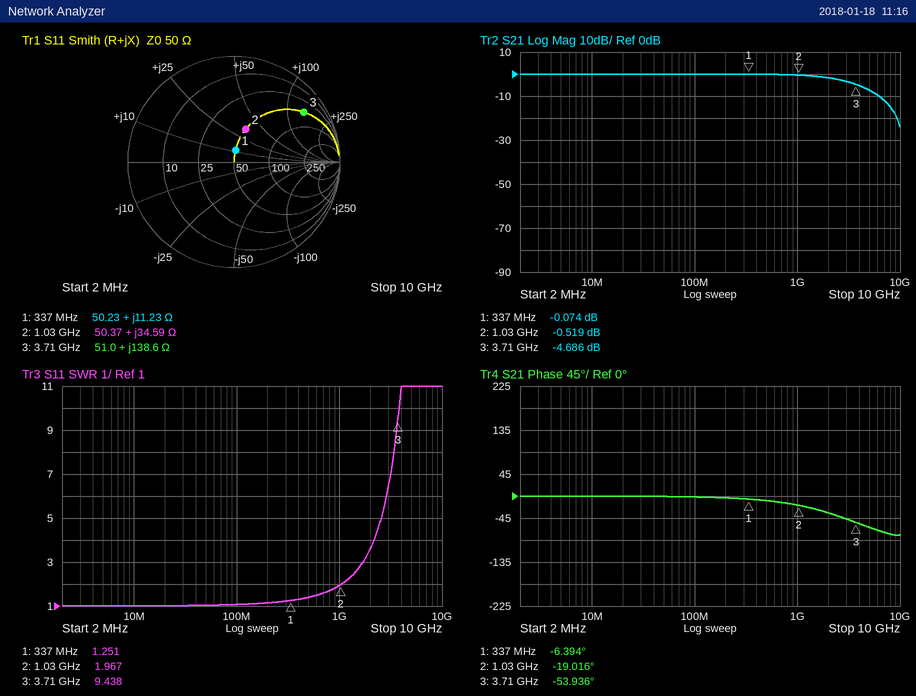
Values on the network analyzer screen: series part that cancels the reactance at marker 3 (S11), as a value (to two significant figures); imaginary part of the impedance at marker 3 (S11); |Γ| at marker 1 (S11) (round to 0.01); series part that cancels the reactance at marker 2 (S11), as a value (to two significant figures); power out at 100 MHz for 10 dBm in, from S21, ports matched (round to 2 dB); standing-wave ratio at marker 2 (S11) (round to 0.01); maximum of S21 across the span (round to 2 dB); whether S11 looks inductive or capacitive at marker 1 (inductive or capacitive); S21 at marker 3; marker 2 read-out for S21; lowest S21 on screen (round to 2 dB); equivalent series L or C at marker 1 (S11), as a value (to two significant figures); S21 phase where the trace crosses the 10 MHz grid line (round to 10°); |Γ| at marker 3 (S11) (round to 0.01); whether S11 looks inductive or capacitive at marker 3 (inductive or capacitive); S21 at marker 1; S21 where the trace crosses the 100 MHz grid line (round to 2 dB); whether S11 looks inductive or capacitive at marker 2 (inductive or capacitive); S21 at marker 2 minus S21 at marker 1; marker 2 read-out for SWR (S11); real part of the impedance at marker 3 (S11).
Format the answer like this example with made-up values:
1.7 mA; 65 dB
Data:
310 fF; +138.6 Ω; 0.11; 4.5 pF; 10 dBm; 1.97; 0 dB; inductive; -4.686 dB; -0.519 dB; -24 dB; 5.3 nH; 0°; 0.81; inductive; -0.074 dB; 0 dB; inductive; -0.445 dB; 1.967; 51.0 Ω
